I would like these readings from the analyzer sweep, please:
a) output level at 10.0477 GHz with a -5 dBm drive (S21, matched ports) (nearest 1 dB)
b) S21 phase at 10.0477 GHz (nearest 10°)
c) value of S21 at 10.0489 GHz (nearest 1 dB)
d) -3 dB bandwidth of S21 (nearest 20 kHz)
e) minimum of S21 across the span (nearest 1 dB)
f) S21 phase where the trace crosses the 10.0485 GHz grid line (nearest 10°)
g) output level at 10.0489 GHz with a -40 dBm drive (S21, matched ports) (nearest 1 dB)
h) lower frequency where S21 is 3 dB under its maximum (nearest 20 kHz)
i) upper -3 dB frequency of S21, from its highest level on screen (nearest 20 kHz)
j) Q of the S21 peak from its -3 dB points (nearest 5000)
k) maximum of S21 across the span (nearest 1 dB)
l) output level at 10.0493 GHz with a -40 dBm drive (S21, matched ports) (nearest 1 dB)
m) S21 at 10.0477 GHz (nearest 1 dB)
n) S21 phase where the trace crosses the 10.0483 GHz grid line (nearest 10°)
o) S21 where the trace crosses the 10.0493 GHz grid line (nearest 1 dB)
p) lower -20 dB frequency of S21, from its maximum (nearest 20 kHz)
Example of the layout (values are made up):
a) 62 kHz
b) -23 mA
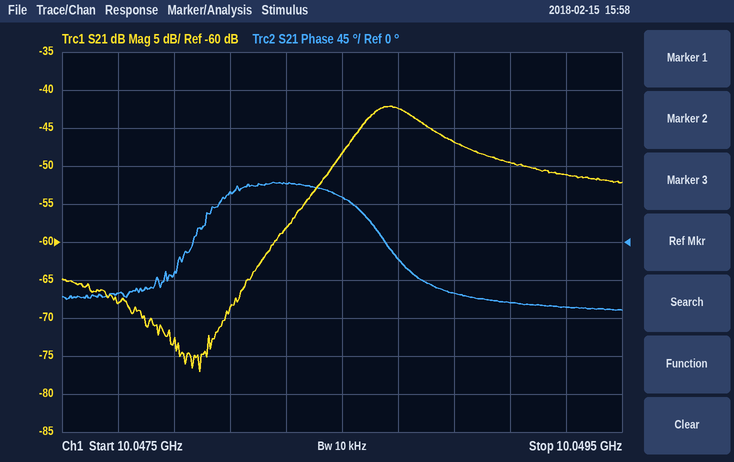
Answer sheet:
a) -73 dBm
b) -60°
c) -47 dB
d) 260 kHz
e) -77 dB
f) 50°
g) -87 dBm
h) 10.04856 GHz
i) 10.04882 GHz
j) 40000
k) -42 dB
l) -91 dBm
m) -68 dB
n) 70°
o) -51 dB
p) 10.04822 GHz
